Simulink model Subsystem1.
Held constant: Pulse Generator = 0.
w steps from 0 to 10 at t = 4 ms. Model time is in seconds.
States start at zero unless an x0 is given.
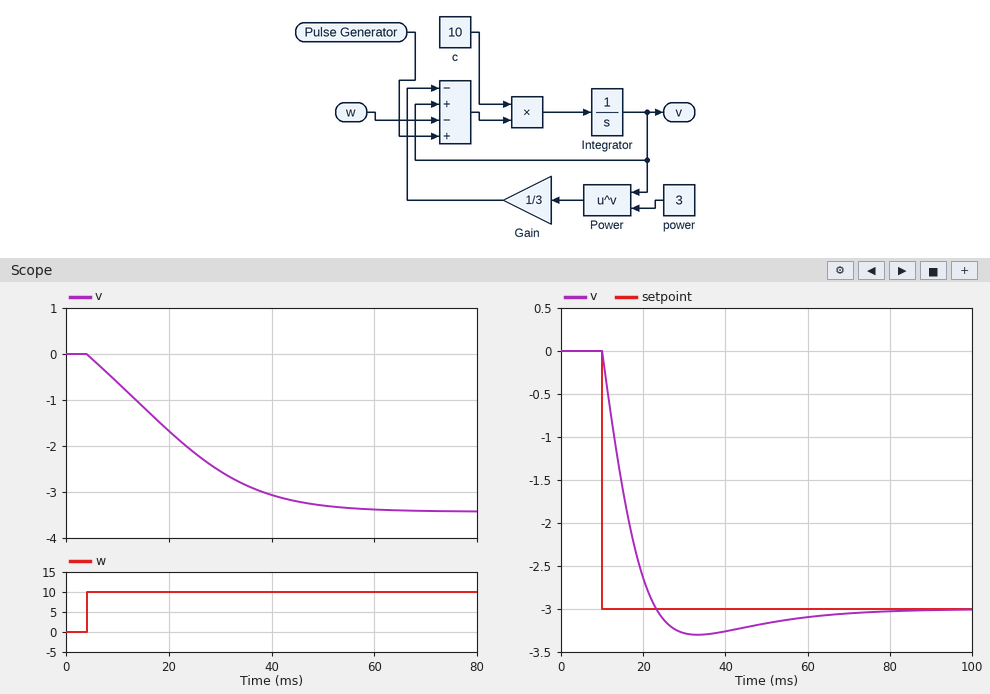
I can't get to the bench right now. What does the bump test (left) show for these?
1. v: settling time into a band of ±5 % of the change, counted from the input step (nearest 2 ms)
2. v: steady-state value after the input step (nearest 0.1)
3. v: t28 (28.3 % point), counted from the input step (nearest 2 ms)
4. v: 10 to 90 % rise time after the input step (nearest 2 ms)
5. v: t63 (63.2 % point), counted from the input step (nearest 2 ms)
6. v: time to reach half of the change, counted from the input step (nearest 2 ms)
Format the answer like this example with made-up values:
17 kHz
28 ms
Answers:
44 ms
-3.4
10 ms
34 ms
22 ms
16 ms
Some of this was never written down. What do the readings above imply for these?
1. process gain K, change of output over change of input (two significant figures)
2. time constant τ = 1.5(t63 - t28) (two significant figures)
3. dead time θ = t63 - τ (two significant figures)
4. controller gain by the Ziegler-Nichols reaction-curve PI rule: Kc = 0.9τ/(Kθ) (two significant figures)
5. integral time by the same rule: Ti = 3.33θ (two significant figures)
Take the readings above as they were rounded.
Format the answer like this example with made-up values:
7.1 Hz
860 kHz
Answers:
-0.34
18 ms
4.0 ms
-12
13 ms
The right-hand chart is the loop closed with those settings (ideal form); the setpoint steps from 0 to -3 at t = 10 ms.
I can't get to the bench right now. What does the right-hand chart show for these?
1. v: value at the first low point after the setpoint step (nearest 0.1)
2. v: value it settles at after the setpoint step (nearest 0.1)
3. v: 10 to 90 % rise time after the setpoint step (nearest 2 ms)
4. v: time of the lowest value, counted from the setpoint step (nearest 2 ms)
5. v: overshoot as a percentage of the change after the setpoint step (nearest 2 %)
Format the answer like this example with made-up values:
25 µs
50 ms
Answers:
-3.3
-3.0
10 ms
24 ms
10 %
